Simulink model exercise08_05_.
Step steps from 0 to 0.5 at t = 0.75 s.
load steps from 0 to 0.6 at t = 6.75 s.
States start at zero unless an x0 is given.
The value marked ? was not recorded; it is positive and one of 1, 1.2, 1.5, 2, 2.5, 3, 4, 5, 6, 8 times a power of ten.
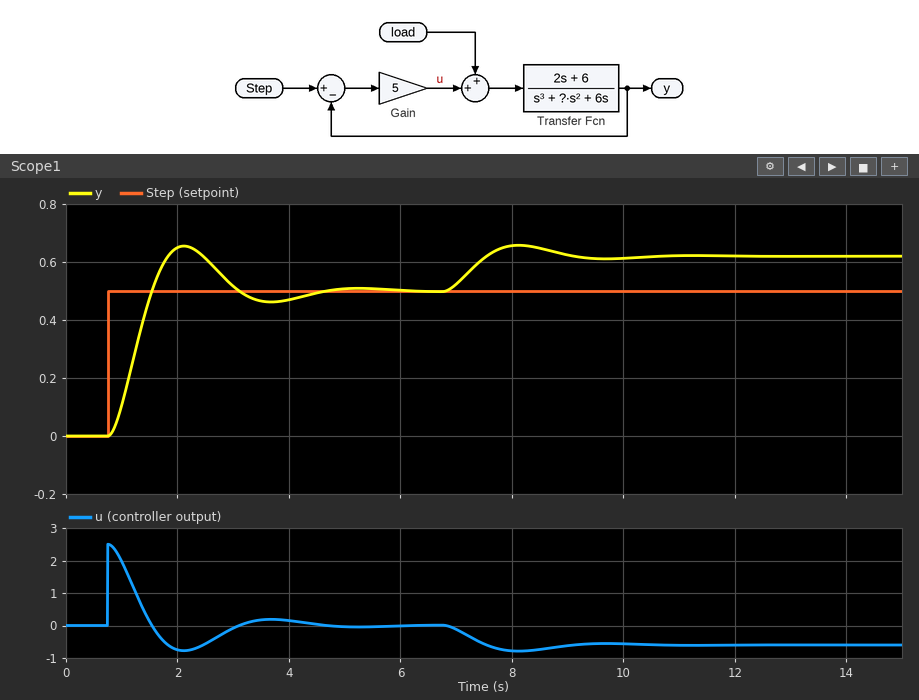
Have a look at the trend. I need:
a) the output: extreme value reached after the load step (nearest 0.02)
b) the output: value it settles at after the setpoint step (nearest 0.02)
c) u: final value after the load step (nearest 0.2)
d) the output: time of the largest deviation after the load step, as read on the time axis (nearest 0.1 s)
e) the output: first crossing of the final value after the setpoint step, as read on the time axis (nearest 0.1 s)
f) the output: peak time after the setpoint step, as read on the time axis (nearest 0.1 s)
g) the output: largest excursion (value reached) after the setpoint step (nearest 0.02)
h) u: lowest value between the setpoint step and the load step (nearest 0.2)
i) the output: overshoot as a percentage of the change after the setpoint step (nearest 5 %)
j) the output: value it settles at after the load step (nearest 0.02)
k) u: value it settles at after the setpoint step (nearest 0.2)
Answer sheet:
0.66
0.50
-0.6
8.1 s
1.5 s
2.1 s
0.66
-0.8
30 %
0.62
0.0
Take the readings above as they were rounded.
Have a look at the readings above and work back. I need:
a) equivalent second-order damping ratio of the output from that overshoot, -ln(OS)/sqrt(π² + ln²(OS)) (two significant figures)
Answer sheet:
0.36
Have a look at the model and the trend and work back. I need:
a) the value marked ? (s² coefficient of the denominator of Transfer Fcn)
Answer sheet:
8
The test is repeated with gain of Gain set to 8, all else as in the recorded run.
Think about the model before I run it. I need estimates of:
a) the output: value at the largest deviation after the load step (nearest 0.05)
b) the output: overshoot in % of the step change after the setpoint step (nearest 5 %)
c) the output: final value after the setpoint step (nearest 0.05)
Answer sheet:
0.60
35 %
0.50
